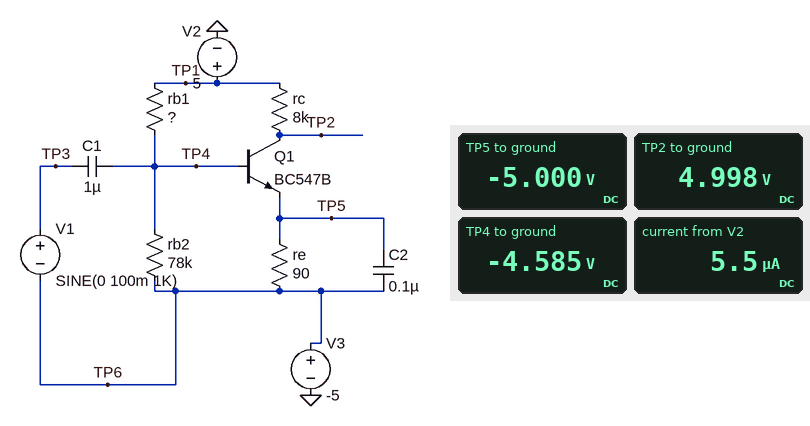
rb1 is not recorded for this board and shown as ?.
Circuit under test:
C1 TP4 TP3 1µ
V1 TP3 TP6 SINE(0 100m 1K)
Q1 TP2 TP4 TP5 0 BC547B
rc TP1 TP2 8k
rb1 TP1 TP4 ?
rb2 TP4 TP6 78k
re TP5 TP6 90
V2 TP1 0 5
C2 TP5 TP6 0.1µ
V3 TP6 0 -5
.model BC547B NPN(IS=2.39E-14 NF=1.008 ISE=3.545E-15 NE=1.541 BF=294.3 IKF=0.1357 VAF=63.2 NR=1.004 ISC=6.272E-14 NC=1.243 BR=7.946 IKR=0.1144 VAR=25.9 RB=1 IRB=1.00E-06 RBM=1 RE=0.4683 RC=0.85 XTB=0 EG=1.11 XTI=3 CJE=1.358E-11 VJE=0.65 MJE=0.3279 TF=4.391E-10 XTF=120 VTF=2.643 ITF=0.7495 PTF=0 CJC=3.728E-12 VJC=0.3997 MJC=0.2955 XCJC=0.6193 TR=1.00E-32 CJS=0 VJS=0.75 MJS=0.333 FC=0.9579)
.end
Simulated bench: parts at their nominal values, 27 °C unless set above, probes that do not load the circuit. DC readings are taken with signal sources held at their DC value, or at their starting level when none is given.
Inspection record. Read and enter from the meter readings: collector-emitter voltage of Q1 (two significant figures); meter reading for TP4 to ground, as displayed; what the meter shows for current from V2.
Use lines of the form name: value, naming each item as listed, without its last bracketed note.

collector-emitter voltage of Q1: 10 V
meter reading for TP4 to ground, as displayed: -4.585 V
what the meter shows for current from V2: 5.5 µA
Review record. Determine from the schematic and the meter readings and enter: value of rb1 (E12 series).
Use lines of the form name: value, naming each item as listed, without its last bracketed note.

value of rb1: 1.8 MΩ
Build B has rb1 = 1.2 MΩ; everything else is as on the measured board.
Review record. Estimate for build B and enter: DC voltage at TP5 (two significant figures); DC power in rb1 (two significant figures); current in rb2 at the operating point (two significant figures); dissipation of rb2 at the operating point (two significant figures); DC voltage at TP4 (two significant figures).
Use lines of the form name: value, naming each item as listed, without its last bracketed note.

DC voltage at TP5: -5.0 V
DC power in rb1: 74 µW
current in rb2 at the operating point: 7.5 µA
dissipation of rb2 at the operating point: 4.4 µW
DC voltage at TP4: -4.4 V
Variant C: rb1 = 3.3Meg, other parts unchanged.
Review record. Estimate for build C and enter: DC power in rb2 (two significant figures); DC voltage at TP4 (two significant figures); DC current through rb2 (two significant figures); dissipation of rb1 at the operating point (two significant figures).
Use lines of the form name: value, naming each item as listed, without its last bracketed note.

DC power in rb2: 680 nW
DC voltage at TP4: -4.8 V
DC current through rb2: 3.0 µA
dissipation of rb1 at the operating point: 29 µW
